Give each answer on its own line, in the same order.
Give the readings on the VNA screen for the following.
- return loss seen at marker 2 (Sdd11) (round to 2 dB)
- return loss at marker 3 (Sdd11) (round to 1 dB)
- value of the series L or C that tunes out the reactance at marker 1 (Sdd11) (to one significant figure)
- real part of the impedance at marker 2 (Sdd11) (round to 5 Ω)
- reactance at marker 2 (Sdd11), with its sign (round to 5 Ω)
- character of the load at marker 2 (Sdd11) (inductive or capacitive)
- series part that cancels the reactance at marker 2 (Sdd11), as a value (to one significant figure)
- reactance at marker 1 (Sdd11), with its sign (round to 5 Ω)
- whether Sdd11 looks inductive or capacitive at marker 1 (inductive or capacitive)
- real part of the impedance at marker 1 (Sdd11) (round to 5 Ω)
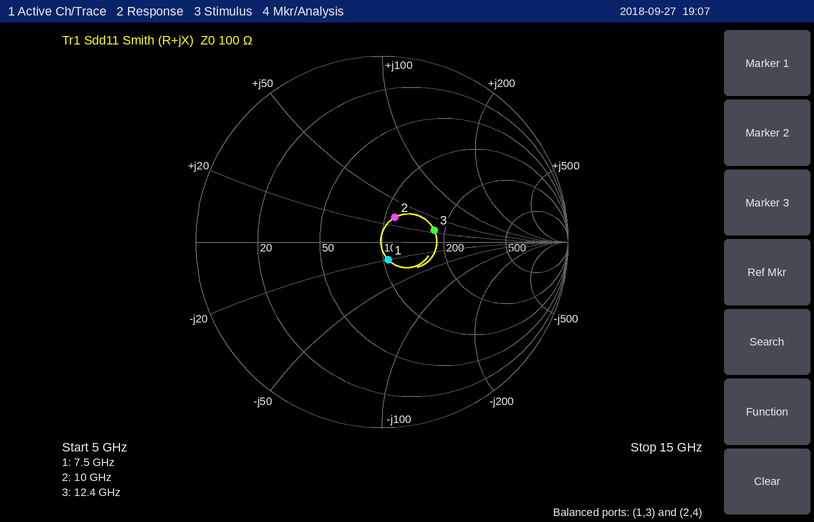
16 dB
11 dB
400 pH
110 Ω
+30 Ω
inductive
500 fF
-20 Ω
capacitive
105 Ω
